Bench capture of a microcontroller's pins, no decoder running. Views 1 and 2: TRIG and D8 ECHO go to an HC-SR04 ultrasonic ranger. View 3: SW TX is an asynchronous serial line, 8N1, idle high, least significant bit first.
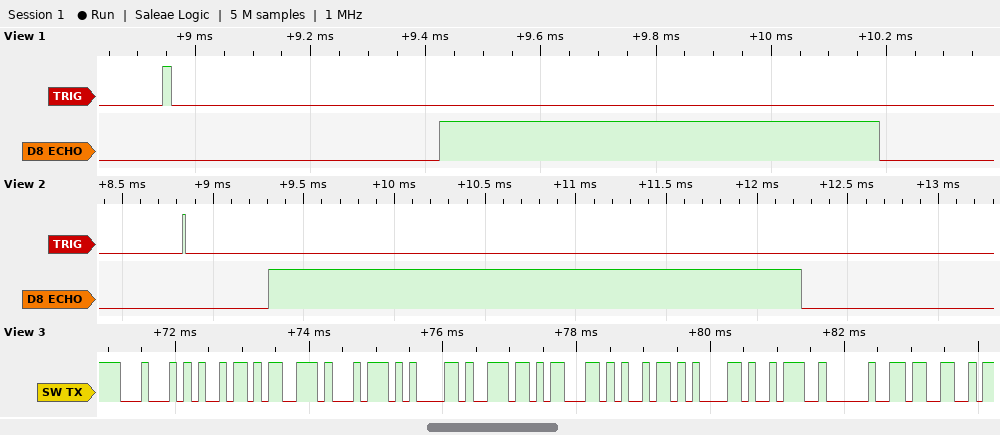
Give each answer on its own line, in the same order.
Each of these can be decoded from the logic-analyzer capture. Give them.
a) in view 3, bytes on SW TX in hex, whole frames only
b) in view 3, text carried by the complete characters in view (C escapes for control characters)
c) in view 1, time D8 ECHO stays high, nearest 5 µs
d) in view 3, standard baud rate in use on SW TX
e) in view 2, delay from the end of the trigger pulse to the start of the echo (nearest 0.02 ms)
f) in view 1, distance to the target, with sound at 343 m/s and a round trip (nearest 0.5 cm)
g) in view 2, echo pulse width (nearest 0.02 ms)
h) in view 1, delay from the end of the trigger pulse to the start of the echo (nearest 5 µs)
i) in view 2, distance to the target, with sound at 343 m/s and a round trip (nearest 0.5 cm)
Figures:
44 69 73 74 61 6E 63 69 61 3A 20 33
"Distancia: 3"
765 µs
9600 baud
0.46 ms
13 cm
2.94 ms
465 µs
50.5 cm
